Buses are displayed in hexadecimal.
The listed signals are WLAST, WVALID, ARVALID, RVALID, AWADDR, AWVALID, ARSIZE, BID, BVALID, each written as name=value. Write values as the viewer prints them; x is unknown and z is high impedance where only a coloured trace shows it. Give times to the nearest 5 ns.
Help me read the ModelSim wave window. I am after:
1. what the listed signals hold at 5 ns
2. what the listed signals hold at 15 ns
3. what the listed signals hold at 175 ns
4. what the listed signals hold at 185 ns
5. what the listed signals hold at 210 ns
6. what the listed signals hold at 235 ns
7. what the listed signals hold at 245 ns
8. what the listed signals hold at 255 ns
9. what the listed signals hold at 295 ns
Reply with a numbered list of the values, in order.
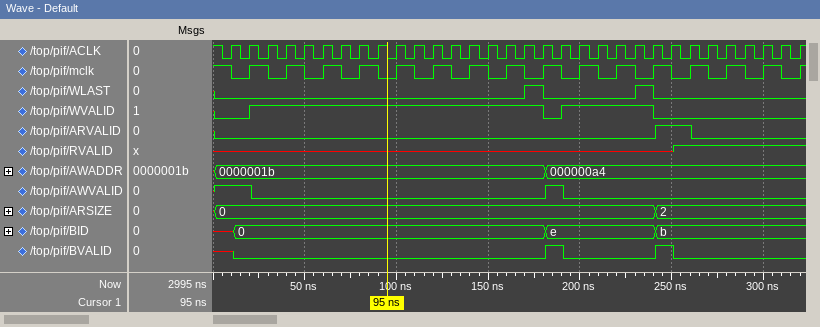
1. WLAST=0, WVALID=0, ARVALID=0, RVALID=x, AWADDR=0000001b, AWVALID=1, ARSIZE=0, BID=x, BVALID=x
2. WLAST=0, WVALID=0, ARVALID=0, RVALID=x, AWADDR=0000001b, AWVALID=1, ARSIZE=0, BID=0, BVALID=0
3. WLAST=1, WVALID=1, ARVALID=0, RVALID=x, AWADDR=0000001b, AWVALID=0, ARSIZE=0, BID=0, BVALID=0
4. WLAST=0, WVALID=0, ARVALID=0, RVALID=x, AWADDR=000000a4, AWVALID=1, ARSIZE=0, BID=e, BVALID=1
5. WLAST=0, WVALID=1, ARVALID=0, RVALID=x, AWADDR=000000a4, AWVALID=0, ARSIZE=0, BID=e, BVALID=0
6. WLAST=1, WVALID=1, ARVALID=0, RVALID=x, AWADDR=000000a4, AWVALID=0, ARSIZE=0, BID=e, BVALID=0
7. WLAST=0, WVALID=0, ARVALID=1, RVALID=x, AWADDR=000000a4, AWVALID=0, ARSIZE=2, BID=b, BVALID=1
8. WLAST=0, WVALID=0, ARVALID=1, RVALID=1, AWADDR=000000a4, AWVALID=0, ARSIZE=2, BID=b, BVALID=0
9. WLAST=0, WVALID=0, ARVALID=0, RVALID=1, AWADDR=000000a4, AWVALID=0, ARSIZE=2, BID=b, BVALID=0
